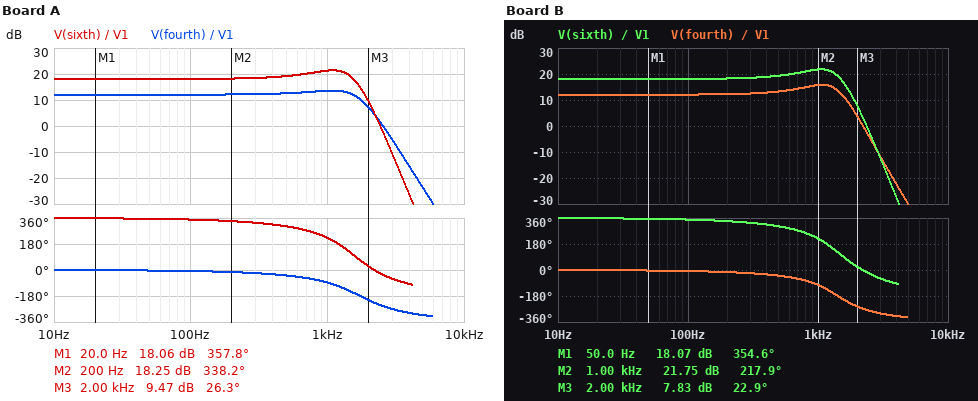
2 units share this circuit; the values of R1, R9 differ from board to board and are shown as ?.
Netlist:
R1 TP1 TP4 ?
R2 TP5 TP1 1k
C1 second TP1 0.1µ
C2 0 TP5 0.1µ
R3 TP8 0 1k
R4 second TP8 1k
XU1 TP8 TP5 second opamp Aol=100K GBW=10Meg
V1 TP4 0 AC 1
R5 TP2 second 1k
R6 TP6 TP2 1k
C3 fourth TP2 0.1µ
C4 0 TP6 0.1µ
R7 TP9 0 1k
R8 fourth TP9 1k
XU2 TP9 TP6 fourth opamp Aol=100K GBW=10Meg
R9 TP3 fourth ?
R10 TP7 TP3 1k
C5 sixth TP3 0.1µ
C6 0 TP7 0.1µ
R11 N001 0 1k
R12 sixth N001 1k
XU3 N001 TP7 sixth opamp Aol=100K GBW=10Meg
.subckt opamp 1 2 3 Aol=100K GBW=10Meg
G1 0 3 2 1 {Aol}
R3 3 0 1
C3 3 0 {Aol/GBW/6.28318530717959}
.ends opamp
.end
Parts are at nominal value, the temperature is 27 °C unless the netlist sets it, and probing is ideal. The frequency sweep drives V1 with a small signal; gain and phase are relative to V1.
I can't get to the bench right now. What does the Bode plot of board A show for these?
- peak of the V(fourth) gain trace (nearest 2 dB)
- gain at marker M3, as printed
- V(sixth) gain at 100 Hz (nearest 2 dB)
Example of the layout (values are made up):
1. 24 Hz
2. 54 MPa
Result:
1. 14 dB
2. 9.47 dB
3. 18 dB
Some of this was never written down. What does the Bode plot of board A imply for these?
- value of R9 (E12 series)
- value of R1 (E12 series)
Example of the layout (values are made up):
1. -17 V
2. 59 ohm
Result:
1. 1.2 kΩ
2. 680 Ω
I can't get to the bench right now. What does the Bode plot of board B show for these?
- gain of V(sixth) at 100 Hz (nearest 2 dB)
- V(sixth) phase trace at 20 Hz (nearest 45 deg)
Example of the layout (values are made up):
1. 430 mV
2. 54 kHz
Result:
1. 18 dB
2. 360 deg
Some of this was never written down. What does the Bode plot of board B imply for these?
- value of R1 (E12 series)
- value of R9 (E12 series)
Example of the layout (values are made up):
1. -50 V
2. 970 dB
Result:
1. 1.5 kΩ
2. 560 Ω
